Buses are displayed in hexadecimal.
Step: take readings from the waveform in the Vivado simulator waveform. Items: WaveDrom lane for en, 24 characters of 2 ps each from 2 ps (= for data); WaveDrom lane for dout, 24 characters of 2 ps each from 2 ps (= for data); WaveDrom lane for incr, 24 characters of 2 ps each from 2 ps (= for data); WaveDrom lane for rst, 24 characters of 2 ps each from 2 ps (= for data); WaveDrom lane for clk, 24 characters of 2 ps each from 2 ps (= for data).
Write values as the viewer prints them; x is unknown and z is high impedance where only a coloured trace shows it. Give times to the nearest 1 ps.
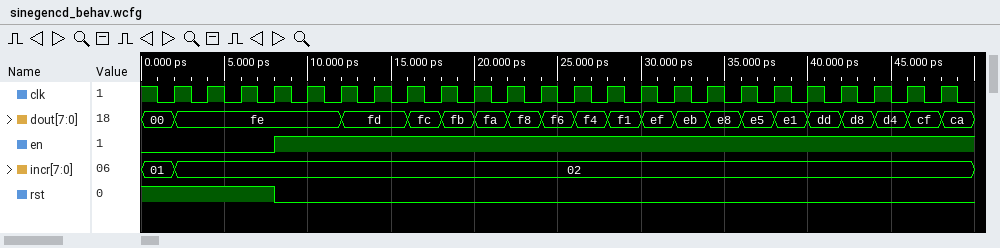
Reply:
{name: 'en', wave: '0..1....................'}
{name: 'dout', wave: '=....=.=================', data: 'fe fd fc fb fa f8 f6 f4 f1 ef eb e8 e5 e1 dd d8 d4 cf ca'}
{name: 'incr', wave: '=.......................', data: '02'}
{name: 'rst', wave: '1..0....................'}
{name: 'clk', wave: 'p.......................'}
